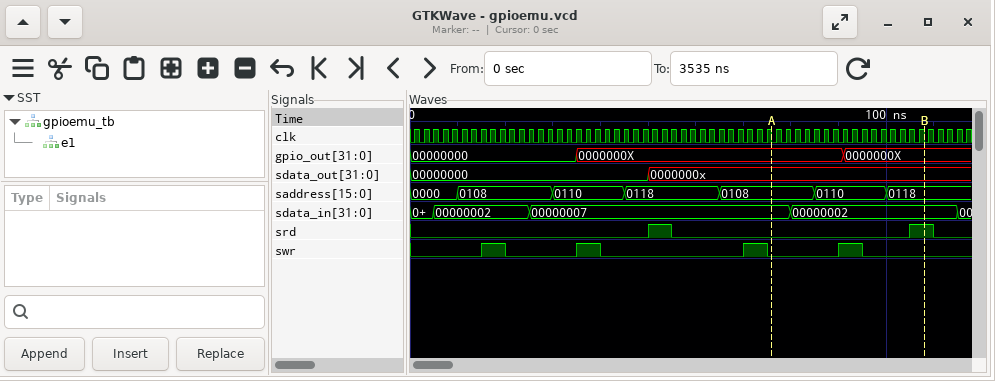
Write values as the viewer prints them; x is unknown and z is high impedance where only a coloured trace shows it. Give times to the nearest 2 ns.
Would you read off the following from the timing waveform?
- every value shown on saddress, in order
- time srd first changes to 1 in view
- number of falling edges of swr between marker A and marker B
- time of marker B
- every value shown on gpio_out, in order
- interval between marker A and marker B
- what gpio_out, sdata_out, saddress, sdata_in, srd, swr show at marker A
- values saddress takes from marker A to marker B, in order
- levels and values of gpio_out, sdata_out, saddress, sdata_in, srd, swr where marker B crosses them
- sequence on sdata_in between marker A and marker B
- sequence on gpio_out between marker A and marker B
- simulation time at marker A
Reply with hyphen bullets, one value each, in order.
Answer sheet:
- 0000, 0108, 0110, 0118, 0108, 0110, 0118
- 50 ns
- 1
- 108 ns
- 00000000, 0000000X, 0000000X
- 32 ns
- gpio_out=0000000X, sdata_out=0000000x, saddress=0108, sdata_in=00000007, srd=0, swr=0
- 0108, 0110, 0118
- gpio_out=0000000X, sdata_out=0000000x, saddress=0118, sdata_in=00000002, srd=1, swr=0
- 00000007, 00000002
- 0000000X, 0000000X
- 76 ns
